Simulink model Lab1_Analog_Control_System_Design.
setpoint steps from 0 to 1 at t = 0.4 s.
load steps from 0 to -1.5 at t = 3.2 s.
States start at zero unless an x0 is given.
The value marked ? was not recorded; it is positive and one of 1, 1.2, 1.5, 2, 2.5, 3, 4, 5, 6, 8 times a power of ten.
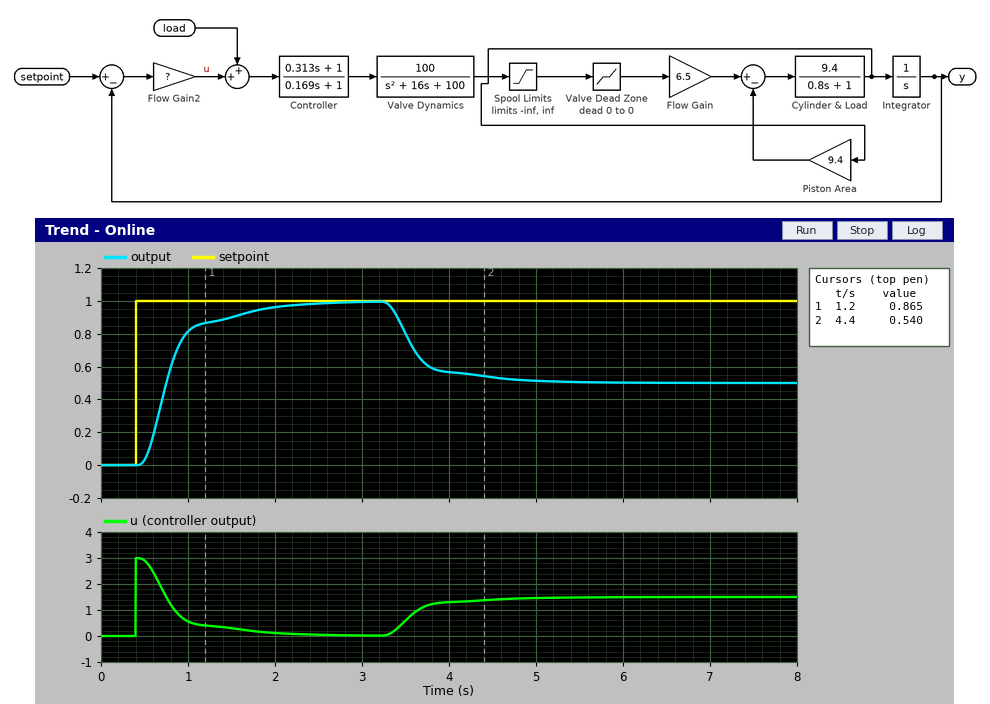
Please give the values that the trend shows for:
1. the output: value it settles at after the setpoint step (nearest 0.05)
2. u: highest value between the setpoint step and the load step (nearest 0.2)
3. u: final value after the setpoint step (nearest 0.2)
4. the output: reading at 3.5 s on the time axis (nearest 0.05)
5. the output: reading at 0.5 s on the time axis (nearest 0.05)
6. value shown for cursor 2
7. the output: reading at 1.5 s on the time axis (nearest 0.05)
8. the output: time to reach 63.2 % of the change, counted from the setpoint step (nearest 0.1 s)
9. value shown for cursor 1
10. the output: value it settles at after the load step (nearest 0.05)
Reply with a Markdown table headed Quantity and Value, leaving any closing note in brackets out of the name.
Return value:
| Quantity | Value |
|---|---|
| the output: value it settles at after the setpoint step | 1.00 |
| u: highest value between the setpoint step and the load step | 3.0 |
| u: final value after the setpoint step | 0.0 |
| the output: reading at 3.5 s on the time axis | 0.80 |
| the output: reading at 0.5 s on the time axis | 0.05 |
| value shown for cursor 2 | 0.540 |
| the output: reading at 1.5 s on the time axis | 0.90 |
| the output: time to reach 63.2 % of the change, counted from the setpoint step | 0.4 s |
| value shown for cursor 1 | 0.865 |
| the output: value it settles at after the load step | 0.50 |
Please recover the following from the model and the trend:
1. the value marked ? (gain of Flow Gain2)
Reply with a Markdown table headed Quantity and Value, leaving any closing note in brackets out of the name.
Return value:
| Quantity | Value |
|---|---|
| the value marked ? | 3 |
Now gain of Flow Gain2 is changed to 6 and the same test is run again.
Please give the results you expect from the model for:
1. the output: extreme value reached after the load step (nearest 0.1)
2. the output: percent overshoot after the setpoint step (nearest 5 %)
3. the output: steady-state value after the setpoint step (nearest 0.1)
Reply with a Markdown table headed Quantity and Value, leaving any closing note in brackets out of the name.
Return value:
| Quantity | Value |
|---|---|
| the output: extreme value reached after the load step | 0.7 |
| the output: percent overshoot after the setpoint step | 15 % |
| the output: steady-state value after the setpoint step | 1.0 |
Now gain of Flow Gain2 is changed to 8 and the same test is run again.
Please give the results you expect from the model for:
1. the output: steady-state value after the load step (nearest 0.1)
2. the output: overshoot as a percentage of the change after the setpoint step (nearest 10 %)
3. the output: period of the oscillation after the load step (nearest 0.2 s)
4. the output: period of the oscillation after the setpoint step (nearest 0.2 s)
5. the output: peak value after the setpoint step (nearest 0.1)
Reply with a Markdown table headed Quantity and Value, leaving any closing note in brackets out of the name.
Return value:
| Quantity | Value |
|---|---|
| the output: steady-state value after the load step | 0.8 |
| the output: overshoot as a percentage of the change after the setpoint step | 30 % |
| the output: period of the oscillation after the load step | 0.8 s |
| the output: period of the oscillation after the setpoint step | 0.8 s |
| the output: peak value after the setpoint step | 1.3 |
